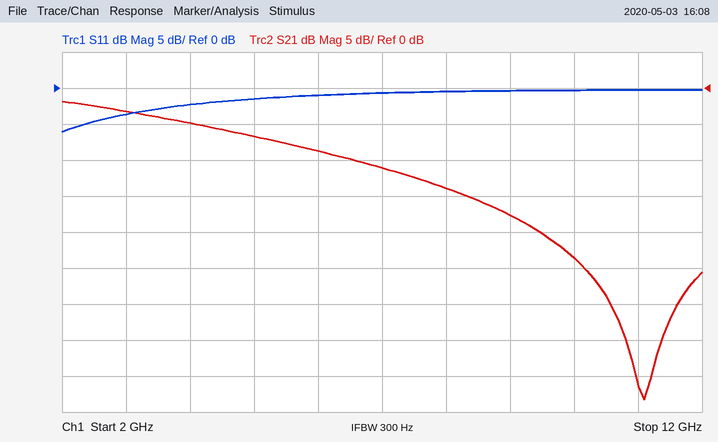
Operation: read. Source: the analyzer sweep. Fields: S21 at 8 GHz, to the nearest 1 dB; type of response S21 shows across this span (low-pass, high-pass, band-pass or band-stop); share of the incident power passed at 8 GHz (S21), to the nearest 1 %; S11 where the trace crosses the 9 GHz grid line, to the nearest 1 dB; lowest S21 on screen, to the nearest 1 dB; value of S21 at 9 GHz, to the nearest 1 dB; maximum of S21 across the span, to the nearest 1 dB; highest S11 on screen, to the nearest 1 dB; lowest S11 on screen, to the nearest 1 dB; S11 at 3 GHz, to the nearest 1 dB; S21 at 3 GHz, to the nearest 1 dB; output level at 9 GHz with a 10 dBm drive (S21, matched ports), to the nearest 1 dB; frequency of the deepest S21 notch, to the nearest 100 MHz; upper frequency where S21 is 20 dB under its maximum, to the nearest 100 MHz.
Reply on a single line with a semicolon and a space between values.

-14 dB; low-pass; 4 %; 0 dB; -43 dB; -18 dB; -2 dB; 0 dB; -6 dB; -4 dB; -3 dB; -8 dBm; 11.1 GHz; 9.8 GHz
